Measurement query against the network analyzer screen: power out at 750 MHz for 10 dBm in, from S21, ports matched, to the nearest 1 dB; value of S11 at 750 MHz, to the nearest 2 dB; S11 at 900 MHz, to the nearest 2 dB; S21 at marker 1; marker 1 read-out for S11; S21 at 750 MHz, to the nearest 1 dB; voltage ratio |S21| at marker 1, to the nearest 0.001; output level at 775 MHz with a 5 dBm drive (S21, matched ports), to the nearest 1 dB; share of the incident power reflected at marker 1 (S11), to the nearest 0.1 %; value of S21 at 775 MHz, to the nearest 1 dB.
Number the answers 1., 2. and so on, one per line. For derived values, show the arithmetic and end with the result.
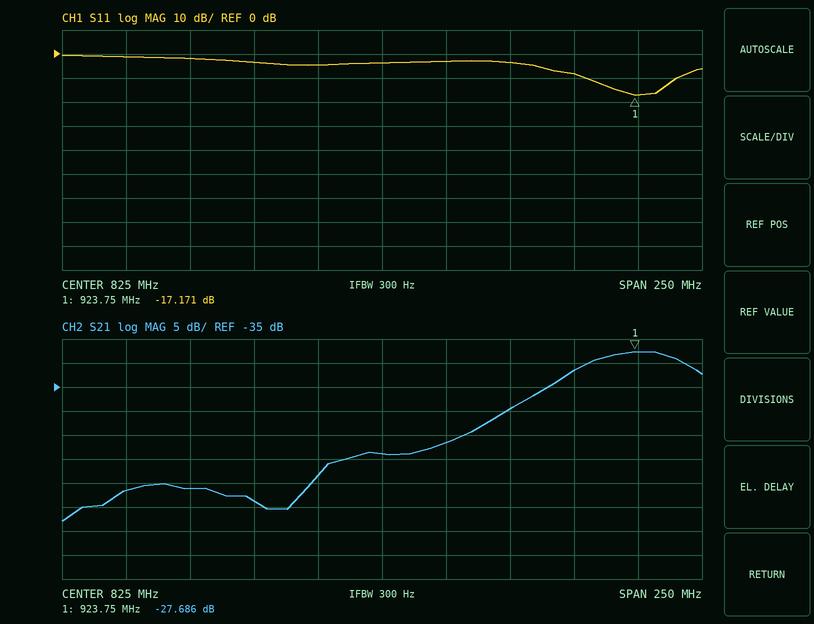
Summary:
1. 10 dBm + (-56 dB) = -46 dBm
2. -2 dB
3. -8 dB
4. -27.686 dB
5. -17.171 dB
6. -56 dB
7. 10^(-27.686/20) ≈ 0.041
8. 5 dBm + (-59 dB) = -54 dBm
9. 10^(-17.171/10) ≈ 1.9 %
10. -59 dB
